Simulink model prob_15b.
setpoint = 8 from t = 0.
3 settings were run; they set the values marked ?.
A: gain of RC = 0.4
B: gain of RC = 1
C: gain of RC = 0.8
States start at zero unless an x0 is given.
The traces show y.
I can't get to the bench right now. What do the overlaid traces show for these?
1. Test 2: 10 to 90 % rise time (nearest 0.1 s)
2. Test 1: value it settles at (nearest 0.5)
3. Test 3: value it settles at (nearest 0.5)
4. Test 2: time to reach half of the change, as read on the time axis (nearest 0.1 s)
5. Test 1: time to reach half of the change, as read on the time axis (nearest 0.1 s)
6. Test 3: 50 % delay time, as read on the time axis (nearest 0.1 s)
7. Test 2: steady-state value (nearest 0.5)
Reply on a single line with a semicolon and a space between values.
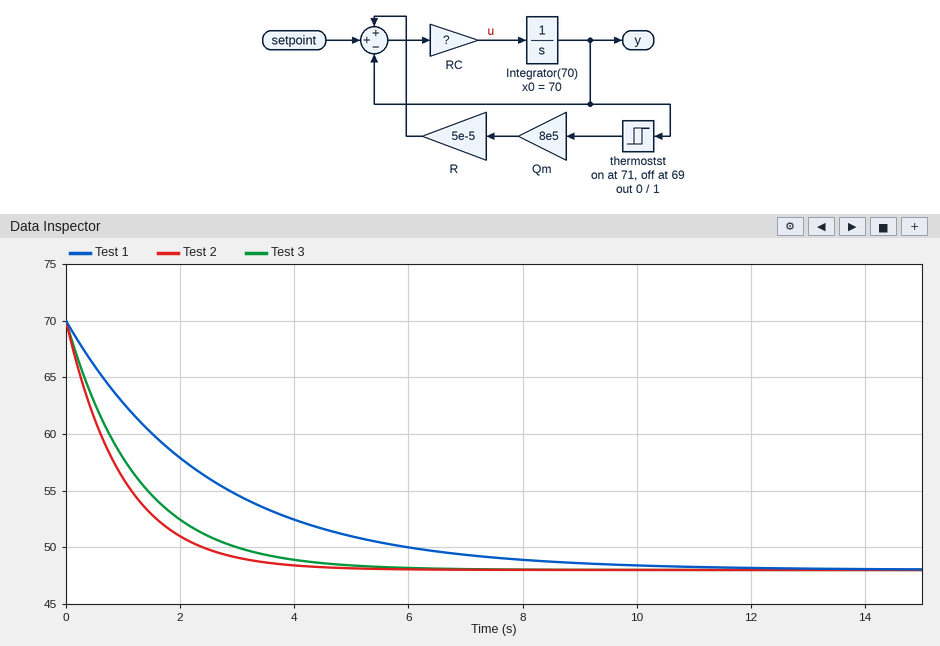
2.2 s; 48.0; 48.0; 0.7 s; 1.7 s; 0.9 s; 48.0
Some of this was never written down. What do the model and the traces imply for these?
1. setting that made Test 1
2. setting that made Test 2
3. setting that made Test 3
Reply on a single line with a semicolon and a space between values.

A; B; C
